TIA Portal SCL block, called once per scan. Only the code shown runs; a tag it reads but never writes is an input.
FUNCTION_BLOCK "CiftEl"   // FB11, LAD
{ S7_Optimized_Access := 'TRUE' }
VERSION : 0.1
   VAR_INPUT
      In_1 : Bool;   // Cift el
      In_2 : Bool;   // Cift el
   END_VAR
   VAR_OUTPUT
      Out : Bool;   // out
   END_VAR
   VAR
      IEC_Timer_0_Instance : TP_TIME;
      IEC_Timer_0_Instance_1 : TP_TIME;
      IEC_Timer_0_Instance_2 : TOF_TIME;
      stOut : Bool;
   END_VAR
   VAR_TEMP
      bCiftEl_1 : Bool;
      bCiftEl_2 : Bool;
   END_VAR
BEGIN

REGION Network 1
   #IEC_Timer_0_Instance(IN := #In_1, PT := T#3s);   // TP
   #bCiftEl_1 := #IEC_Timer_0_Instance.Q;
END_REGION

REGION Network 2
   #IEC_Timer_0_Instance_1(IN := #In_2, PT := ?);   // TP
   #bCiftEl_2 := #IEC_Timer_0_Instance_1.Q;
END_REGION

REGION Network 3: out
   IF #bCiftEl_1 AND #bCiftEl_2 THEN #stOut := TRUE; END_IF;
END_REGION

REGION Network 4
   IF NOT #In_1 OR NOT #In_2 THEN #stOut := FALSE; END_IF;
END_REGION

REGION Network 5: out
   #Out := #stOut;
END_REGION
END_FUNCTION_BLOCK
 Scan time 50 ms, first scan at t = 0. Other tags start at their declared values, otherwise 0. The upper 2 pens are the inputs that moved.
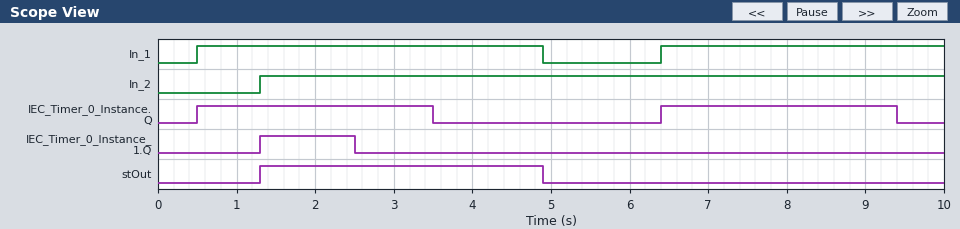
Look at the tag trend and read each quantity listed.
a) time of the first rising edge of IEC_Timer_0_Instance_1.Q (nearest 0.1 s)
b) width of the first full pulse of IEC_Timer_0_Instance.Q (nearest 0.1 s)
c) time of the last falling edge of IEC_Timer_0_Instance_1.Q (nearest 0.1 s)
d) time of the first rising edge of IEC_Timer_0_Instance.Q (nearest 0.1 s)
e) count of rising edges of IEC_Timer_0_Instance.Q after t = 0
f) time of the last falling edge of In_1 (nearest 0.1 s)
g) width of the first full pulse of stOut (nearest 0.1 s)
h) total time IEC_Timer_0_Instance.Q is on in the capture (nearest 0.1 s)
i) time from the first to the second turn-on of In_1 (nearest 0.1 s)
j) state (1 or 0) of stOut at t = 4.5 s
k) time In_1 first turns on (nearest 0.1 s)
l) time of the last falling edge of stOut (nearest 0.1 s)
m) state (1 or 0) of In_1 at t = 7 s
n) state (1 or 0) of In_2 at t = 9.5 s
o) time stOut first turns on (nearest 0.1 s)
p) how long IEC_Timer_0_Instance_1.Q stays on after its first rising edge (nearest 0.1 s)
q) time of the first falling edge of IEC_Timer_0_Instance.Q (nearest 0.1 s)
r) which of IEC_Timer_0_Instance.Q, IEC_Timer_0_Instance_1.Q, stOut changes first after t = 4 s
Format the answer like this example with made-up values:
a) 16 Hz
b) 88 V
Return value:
a) 1.3 s
b) 3.0 s
c) 2.5 s
d) 0.5 s
e) 2
f) 4.9 s
g) 3.6 s
h) 6.0 s
i) 5.9 s
j) 1
k) 0.5 s
l) 4.9 s
m) 1
n) 1
o) 1.3 s
p) 1.2 s
q) 3.5 s
r) stOut
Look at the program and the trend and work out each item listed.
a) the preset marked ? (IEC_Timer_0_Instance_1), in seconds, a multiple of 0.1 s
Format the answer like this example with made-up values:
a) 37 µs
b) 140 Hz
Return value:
a) 1.2 s
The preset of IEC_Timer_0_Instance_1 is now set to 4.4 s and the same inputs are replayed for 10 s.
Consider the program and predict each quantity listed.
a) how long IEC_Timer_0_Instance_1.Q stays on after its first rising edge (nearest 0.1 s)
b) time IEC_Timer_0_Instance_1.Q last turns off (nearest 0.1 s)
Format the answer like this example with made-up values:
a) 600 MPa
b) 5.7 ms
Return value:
a) 4.4 s
b) 5.7 s
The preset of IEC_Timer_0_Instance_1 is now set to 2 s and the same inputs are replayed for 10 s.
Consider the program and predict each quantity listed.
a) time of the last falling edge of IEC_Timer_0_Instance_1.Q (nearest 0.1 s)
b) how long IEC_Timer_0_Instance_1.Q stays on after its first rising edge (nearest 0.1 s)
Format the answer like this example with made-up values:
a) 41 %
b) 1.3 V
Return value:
a) 3.3 s
b) 2.0 s
